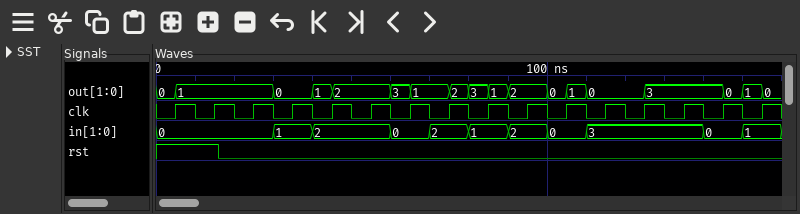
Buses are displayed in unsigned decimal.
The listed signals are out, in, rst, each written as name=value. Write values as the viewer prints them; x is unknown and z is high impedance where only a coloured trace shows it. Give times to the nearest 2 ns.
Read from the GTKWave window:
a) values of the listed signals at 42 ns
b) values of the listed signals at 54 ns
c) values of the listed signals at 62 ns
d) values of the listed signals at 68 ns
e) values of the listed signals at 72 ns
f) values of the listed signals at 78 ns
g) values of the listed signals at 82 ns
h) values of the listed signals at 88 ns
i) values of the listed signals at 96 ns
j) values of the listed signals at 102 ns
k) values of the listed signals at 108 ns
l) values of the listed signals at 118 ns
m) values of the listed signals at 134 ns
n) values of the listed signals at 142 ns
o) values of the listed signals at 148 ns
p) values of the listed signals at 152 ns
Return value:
out=1, in=2, rst=0
out=2, in=2, rst=0
out=3, in=0, rst=0
out=1, in=0, rst=0
out=1, in=2, rst=0
out=2, in=2, rst=0
out=3, in=1, rst=0
out=1, in=1, rst=0
out=2, in=2, rst=0
out=0, in=0, rst=0
out=1, in=0, rst=0
out=0, in=3, rst=0
out=3, in=3, rst=0
out=3, in=0, rst=0
out=0, in=0, rst=0
out=1, in=1, rst=0
